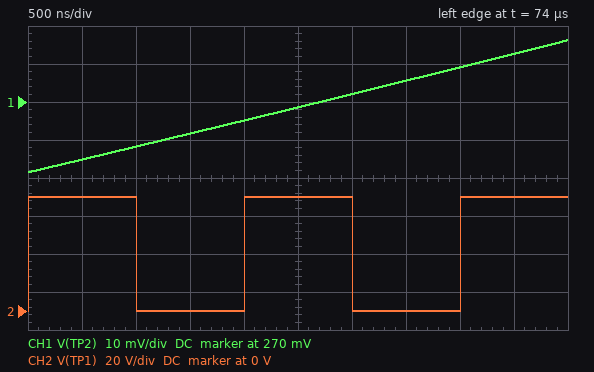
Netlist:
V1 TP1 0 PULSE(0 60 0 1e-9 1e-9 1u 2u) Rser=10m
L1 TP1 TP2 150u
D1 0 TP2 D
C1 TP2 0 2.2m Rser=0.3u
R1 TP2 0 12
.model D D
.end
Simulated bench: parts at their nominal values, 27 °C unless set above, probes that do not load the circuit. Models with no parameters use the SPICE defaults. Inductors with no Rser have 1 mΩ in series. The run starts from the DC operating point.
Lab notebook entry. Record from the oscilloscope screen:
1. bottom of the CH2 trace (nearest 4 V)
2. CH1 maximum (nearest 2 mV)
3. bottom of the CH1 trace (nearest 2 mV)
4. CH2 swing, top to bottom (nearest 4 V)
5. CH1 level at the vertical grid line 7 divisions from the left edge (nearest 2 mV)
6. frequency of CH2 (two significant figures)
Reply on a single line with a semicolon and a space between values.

0 V; 286 mV; 252 mV; 60 V; 276 mV; 500 kHz
